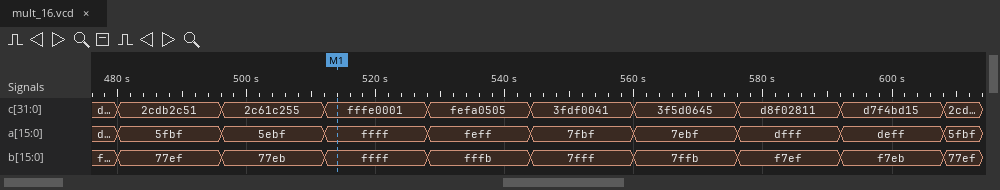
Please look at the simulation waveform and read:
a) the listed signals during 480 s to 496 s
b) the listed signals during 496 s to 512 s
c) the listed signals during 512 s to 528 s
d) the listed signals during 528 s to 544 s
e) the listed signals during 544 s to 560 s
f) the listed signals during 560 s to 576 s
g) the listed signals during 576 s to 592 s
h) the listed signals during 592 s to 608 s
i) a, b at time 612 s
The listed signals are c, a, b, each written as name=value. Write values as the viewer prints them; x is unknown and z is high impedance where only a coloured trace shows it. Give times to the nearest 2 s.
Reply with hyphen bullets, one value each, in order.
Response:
- c=2cdb2c51, a=5fbf, b=77ef
- c=2c61c255, a=5ebf, b=77eb
- c=fffe0001, a=ffff, b=ffff
- c=fefa0505, a=feff, b=fffb
- c=3fdf0041, a=7fbf, b=7fff
- c=3f5d0645, a=7ebf, b=7ffb
- c=d8f02811, a=dfff, b=f7ef
- c=d7f4bd15, a=deff, b=f7eb
- a=5fbf, b=77ef
